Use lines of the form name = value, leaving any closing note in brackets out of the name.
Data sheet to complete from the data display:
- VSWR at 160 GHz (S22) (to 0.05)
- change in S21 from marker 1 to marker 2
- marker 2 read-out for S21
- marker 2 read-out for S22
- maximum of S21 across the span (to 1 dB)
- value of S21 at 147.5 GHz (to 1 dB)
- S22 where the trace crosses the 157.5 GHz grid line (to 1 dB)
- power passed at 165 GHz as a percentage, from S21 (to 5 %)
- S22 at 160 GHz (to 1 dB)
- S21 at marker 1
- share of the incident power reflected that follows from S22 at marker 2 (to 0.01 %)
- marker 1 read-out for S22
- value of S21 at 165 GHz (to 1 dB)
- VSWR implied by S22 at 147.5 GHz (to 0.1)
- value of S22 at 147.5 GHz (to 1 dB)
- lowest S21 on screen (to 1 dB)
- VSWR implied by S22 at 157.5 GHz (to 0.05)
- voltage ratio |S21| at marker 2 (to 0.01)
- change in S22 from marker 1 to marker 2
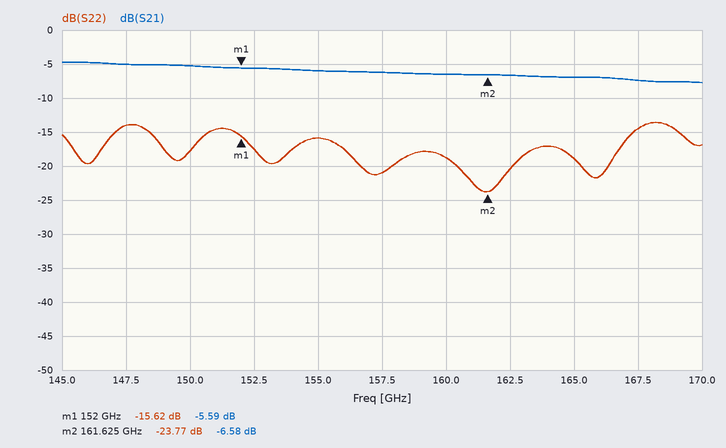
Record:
VSWR at 160 GHz (S22) = 1.25
change in S21 from marker 1 to marker 2 = -0.99 dB
marker 2 read-out for S21 = -6.58 dB
marker 2 read-out for S22 = -23.77 dB
maximum of S21 across the span = -5 dB
value of S21 at 147.5 GHz = -5 dB
S22 where the trace crosses the 157.5 GHz grid line = -21 dB
power passed at 165 GHz as a percentage, from S21 = 20 %
S22 at 160 GHz = -19 dB
S21 at marker 1 = -5.59 dB
share of the incident power reflected that follows from S22 at marker 2 = 0.42 %
marker 1 read-out for S22 = -15.62 dB
value of S21 at 165 GHz = -7 dB
VSWR implied by S22 at 147.5 GHz = 1.5
value of S22 at 147.5 GHz = -14 dB
lowest S21 on screen = -8 dB
VSWR implied by S22 at 157.5 GHz = 1.20
voltage ratio |S21| at marker 2 = 0.47
change in S22 from marker 1 to marker 2 = -8.15 dB
